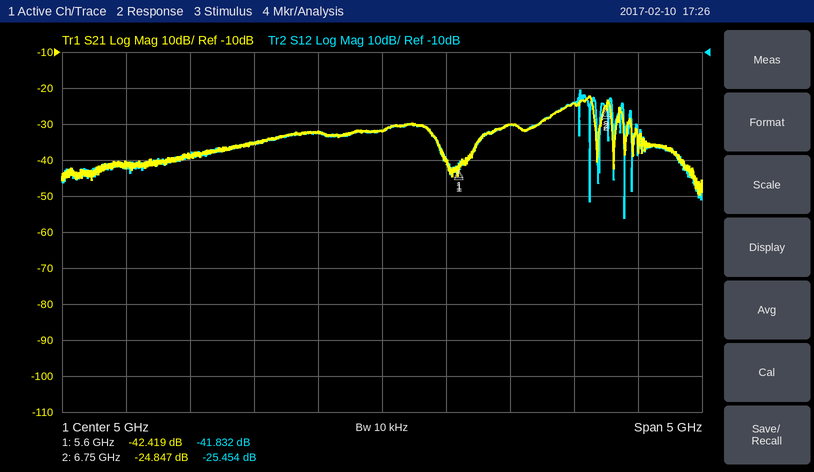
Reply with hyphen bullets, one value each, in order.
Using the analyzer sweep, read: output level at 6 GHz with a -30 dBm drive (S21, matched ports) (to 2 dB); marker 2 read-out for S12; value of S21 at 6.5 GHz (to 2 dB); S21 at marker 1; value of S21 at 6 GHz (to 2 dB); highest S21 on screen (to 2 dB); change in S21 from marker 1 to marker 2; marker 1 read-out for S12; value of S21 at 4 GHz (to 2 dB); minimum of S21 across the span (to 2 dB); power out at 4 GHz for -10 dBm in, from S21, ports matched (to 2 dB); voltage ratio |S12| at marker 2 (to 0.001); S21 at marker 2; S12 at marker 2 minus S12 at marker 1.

- -60 dBm
- -25.454 dB
- -24 dB
- -42.419 dB
- -30 dB
- -22 dB
- 17.572 dB
- -41.832 dB
- -36 dB
- -50 dB
- -46 dBm
- 0.053
- -24.847 dB
- 16.378 dB
